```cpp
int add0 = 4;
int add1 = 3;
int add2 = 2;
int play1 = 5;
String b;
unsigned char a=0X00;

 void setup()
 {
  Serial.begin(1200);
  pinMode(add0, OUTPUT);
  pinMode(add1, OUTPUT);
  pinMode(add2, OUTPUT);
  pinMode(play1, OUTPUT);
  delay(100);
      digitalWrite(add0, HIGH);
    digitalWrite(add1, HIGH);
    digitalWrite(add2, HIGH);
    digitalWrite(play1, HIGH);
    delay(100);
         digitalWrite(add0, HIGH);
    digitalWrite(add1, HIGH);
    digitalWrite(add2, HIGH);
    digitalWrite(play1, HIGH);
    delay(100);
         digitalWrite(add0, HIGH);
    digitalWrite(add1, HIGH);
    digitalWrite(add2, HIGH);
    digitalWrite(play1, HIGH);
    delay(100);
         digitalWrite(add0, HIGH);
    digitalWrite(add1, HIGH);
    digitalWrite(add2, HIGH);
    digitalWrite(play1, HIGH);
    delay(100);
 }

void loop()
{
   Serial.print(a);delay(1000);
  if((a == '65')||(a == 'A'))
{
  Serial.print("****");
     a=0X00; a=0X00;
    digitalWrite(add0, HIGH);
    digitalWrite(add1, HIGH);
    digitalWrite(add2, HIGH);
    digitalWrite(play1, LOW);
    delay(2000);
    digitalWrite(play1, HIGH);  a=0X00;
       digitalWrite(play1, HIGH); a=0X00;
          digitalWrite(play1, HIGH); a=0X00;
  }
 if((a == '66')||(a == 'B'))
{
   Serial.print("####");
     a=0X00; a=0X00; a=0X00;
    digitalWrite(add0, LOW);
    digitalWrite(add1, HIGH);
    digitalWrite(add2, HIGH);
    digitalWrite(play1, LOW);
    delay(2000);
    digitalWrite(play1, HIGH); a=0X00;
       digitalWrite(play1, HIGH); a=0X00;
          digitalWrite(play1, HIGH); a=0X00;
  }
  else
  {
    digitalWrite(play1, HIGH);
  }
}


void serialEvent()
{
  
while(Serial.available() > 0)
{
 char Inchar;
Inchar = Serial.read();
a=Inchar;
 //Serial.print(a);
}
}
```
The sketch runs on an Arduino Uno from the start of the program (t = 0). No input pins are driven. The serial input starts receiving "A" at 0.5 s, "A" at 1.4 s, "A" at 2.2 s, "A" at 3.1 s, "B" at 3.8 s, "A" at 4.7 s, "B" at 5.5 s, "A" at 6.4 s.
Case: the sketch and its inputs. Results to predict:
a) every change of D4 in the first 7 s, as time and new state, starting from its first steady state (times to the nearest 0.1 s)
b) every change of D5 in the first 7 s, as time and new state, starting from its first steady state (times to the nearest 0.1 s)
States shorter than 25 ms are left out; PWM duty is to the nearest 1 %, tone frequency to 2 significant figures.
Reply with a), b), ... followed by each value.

a) 0 s low; 0.1 s high; 5.5 s low
b) 0 s low; 0.1 s high; 2.5 s low; 4.5 s high; 5.5 s low
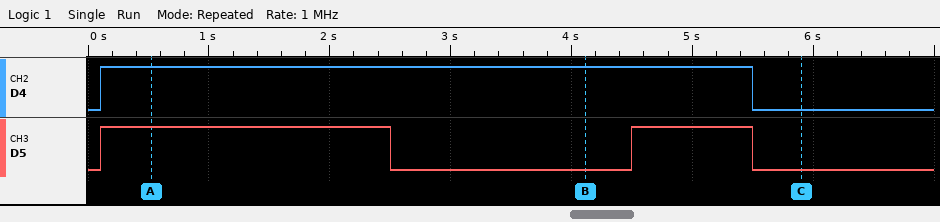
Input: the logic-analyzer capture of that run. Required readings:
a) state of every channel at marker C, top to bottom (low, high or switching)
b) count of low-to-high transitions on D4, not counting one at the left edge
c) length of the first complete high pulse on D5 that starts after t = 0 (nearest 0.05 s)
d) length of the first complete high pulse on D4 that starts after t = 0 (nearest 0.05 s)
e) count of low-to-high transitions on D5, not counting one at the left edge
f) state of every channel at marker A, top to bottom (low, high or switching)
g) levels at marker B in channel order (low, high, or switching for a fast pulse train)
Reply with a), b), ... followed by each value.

a) D4 low, D5 low
b) 1
c) 2.40 s
d) 5.40 s
e) 2
f) D4 high, D5 high
g) D4 high, D5 low
